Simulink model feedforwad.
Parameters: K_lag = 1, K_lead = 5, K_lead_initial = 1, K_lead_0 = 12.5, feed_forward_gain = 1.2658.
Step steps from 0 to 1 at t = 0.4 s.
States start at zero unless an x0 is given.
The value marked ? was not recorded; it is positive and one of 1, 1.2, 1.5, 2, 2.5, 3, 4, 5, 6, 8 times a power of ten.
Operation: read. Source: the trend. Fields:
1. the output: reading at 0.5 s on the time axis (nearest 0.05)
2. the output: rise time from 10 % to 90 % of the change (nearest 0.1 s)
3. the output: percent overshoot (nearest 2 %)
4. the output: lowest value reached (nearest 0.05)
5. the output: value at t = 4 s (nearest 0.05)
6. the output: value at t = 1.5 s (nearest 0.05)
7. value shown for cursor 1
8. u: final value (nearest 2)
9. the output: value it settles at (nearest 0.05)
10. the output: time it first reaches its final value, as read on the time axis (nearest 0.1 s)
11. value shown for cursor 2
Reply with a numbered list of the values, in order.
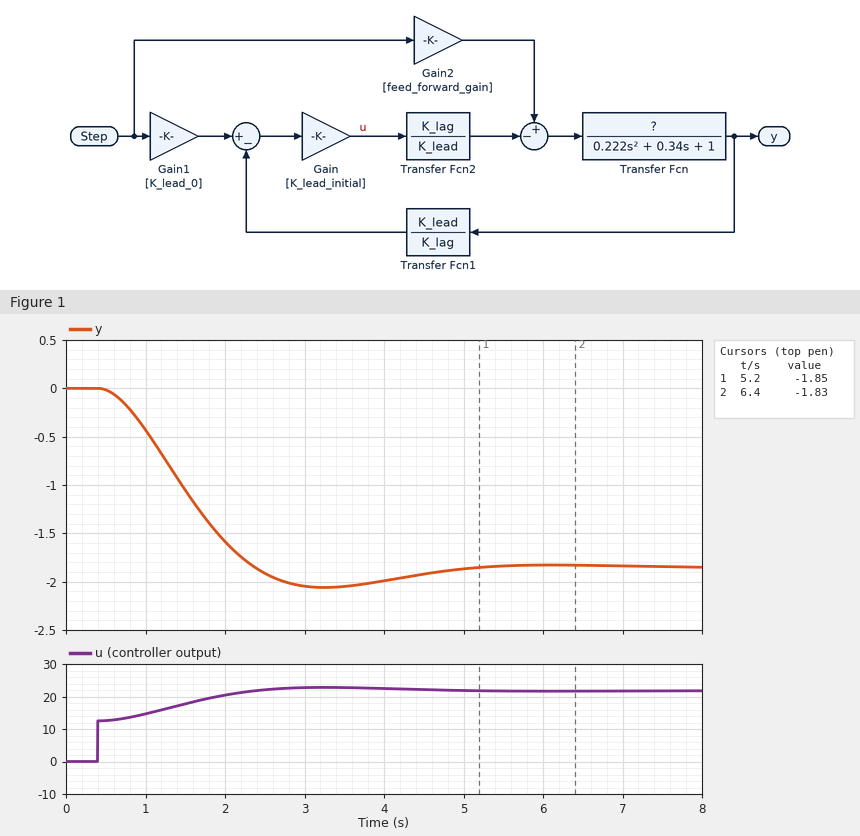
1. 0.00
2. 1.3 s
3. 12 %
4. -2.05
5. -2.00
6. -1.05
7. -1.85
8. 22
9. -1.85
10. 2.4 s
11. -1.83
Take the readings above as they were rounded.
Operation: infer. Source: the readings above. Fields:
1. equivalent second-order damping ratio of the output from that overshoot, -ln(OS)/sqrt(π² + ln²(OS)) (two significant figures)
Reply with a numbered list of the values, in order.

1. 0.56
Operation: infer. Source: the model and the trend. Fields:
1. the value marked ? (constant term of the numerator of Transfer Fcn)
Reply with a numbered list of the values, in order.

1. 0.6
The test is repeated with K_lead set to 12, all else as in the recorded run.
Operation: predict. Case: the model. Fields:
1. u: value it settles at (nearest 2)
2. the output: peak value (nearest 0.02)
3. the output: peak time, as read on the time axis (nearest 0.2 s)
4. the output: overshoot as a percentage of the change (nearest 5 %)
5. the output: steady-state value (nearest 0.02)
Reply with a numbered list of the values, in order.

1. 8
2. 0.38
3. 3.2 s
4. 10 %
5. 0.34
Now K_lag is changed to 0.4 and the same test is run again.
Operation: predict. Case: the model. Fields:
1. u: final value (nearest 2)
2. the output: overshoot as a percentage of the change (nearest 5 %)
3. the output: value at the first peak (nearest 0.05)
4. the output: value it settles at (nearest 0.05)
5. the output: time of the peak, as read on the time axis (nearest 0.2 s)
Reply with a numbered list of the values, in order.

1. 8
2. 10 %
3. 0.45
4. 0.40
5. 3.2 s
